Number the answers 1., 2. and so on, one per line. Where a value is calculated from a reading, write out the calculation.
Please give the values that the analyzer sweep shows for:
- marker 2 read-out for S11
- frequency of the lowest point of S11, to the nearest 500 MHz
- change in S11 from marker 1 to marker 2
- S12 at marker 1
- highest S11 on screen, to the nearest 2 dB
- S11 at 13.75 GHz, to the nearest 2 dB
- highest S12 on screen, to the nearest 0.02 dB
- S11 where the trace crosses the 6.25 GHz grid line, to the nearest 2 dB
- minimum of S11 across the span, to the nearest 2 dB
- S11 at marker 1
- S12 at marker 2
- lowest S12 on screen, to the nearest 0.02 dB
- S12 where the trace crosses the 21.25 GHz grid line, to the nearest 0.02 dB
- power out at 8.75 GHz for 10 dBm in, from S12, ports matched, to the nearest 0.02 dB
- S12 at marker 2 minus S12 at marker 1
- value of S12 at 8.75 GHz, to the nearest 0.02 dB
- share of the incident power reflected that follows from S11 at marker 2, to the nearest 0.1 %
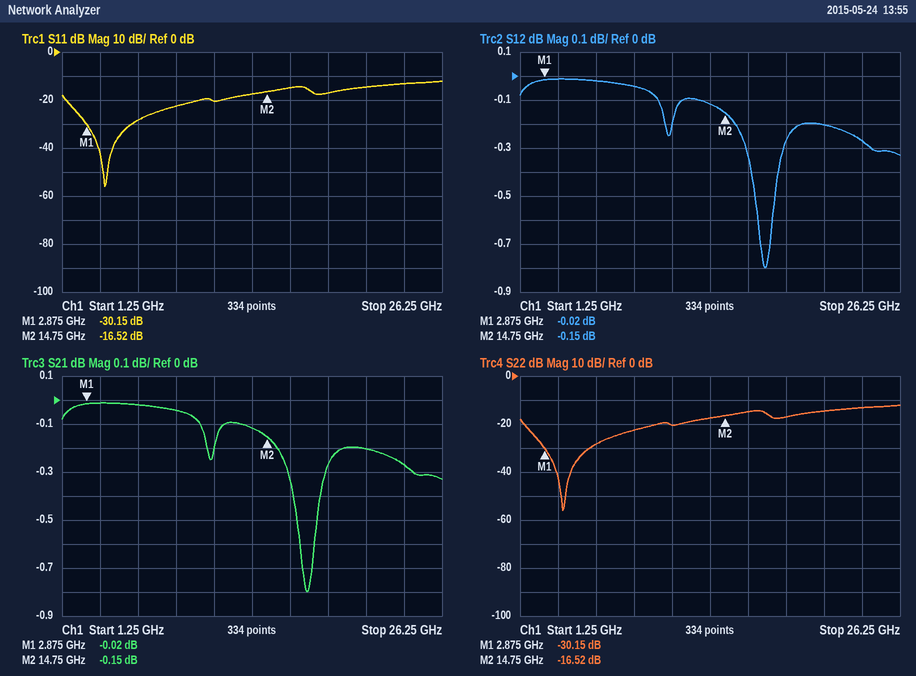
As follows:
1. -16.52 dB
2. 4.0 GHz
3. -16.52 − (-30.15) = 13.63 dB
4. -0.02 dB
5. -12 dB
6. -18 dB
7. -0.02 dB
8. -28 dB
9. -56 dB
10. -30.15 dB
11. -0.15 dB
12. -0.80 dB
13. -0.20 dB
14. 10 dBm + (-0.04 dB) = 9.96 dBm
15. -0.15 − (-0.02) = -0.13 dB
16. -0.04 dB
17. 10^(-16.52/10) ≈ 2.2 %
